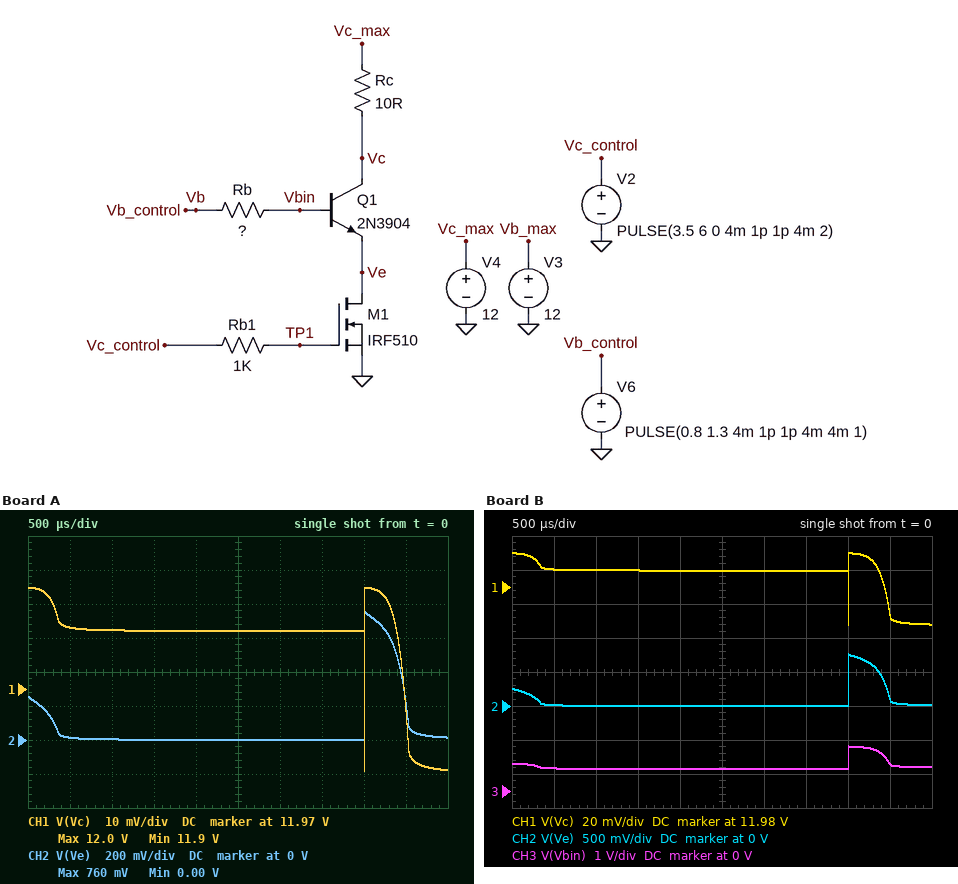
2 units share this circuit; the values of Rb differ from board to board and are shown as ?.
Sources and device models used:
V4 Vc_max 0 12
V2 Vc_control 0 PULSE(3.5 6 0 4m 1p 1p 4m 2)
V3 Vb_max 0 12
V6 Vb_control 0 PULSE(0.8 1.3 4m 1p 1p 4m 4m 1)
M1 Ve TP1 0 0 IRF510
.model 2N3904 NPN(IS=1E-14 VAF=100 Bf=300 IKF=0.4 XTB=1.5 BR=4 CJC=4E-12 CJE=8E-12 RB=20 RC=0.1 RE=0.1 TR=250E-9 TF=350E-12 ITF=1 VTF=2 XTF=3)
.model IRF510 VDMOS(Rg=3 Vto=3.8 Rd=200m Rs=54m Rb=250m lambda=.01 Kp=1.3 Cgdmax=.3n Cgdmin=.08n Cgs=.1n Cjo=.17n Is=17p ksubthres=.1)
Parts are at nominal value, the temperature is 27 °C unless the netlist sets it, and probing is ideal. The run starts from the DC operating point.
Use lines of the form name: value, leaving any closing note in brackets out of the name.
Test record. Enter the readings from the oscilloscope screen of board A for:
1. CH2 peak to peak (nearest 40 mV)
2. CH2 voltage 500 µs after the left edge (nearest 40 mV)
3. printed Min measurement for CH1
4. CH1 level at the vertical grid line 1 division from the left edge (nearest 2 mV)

CH2 peak to peak: 760 mV
CH2 voltage 500 µs after the left edge: 0 V
printed Min measurement for CH1: 11.9 V
CH1 level at the vertical grid line 1 division from the left edge: 11.988 V
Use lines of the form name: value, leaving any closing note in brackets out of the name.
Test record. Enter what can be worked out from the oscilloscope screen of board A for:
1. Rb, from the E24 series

Rb, from the E24 series: 36 kΩ
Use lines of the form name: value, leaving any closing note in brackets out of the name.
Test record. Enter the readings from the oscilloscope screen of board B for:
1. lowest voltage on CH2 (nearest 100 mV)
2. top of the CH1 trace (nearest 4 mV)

lowest voltage on CH2: 0 V
top of the CH1 trace: 12.000 V
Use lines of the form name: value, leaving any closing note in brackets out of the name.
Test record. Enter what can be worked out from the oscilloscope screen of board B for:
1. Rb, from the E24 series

Rb, from the E24 series: 47 kΩ
